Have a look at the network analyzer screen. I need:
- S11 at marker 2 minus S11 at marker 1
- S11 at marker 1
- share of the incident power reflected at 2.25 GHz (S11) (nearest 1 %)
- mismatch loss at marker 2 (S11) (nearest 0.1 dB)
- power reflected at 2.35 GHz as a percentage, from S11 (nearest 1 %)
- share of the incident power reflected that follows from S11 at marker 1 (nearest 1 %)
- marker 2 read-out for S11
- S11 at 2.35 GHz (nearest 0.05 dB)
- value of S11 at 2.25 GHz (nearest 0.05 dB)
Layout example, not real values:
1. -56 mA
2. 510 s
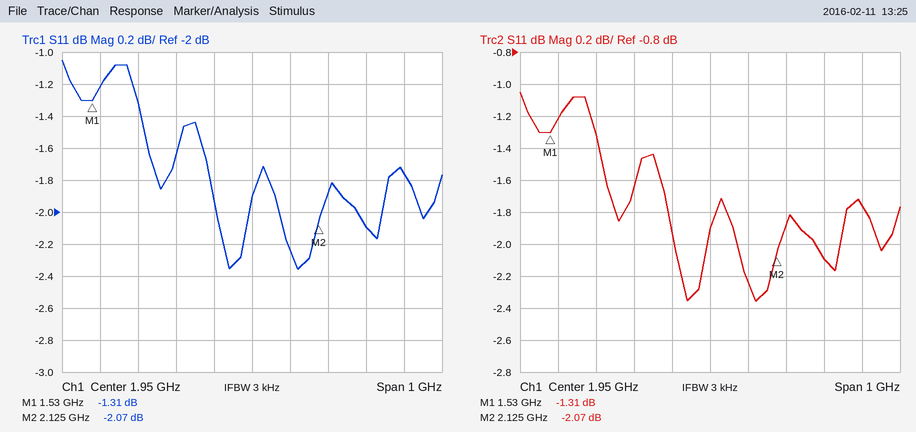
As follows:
1. -0.76 dB
2. -1.31 dB
3. 62 %
4. 4.2 dB
5. 67 %
6. 74 %
7. -2.07 dB
8. -1.75 dB
9. -2.10 dB
